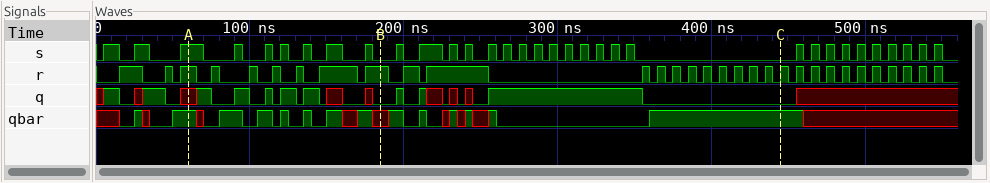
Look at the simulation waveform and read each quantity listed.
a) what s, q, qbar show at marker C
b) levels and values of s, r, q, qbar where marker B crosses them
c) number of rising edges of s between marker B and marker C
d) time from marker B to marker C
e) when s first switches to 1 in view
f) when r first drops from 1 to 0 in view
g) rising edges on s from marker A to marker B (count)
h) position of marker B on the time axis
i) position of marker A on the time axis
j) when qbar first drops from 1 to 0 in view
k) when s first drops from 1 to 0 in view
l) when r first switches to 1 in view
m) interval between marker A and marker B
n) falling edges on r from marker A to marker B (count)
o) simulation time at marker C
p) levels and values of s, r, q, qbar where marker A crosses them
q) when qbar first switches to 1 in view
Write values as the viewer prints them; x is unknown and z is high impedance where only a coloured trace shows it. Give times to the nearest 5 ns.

s=0, q=0, qbar=1
s=0, r=1, q=0, qbar=x
14
260 ns
5 ns
30 ns
6
185 ns
60 ns
95 ns
15 ns
15 ns
125 ns
6
445 ns
s=1, r=1, q=x, qbar=1
25 ns
